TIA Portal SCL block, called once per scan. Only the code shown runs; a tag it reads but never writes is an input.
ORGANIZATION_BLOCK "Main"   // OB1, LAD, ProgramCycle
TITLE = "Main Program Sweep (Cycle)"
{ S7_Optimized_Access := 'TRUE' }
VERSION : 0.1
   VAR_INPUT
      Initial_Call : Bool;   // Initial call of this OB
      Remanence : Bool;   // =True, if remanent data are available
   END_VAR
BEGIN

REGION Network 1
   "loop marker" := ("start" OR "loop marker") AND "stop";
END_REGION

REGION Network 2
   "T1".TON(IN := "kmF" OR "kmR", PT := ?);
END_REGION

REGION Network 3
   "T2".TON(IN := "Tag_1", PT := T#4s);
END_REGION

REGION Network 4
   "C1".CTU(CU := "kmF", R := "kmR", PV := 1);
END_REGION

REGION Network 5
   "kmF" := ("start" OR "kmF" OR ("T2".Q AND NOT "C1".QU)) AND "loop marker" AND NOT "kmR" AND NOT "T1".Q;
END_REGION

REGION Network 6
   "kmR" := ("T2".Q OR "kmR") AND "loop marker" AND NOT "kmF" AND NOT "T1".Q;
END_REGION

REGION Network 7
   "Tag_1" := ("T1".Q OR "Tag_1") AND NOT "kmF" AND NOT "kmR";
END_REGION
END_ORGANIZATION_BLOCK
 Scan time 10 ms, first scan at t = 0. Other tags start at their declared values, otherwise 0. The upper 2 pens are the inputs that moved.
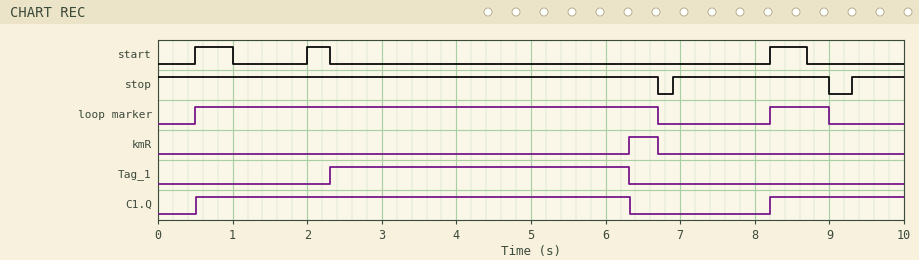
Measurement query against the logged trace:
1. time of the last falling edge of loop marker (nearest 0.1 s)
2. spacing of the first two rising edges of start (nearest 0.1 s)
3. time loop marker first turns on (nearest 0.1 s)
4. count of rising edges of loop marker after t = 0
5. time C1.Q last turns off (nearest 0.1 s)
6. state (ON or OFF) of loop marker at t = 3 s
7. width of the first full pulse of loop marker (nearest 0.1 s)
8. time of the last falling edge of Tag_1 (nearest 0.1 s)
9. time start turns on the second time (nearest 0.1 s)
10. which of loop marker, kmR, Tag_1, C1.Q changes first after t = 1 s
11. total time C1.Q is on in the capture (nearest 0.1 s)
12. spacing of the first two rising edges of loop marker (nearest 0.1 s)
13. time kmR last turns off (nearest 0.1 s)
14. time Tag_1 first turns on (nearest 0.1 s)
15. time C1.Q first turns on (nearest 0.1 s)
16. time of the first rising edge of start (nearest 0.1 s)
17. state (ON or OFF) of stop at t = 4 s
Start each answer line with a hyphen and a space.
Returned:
- 9.0 s
- 1.5 s
- 0.5 s
- 2
- 6.3 s
- ON
- 6.2 s
- 6.3 s
- 2.0 s
- Tag_1
- 7.6 s
- 7.7 s
- 6.7 s
- 2.3 s
- 0.5 s
- 0.5 s
- ON
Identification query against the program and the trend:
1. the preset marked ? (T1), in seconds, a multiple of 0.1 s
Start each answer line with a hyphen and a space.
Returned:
- 1.8 s
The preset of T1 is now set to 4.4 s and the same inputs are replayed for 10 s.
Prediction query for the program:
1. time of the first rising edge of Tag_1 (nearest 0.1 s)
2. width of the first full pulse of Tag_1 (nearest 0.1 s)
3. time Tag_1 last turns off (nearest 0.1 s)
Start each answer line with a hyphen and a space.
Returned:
- 4.9 s
- 3.3 s
- 8.2 s
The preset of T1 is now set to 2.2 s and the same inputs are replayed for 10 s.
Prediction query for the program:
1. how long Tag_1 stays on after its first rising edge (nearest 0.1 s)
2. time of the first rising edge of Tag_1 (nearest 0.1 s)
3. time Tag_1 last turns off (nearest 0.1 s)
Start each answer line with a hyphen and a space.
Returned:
- 5.5 s
- 2.7 s
- 8.2 s
